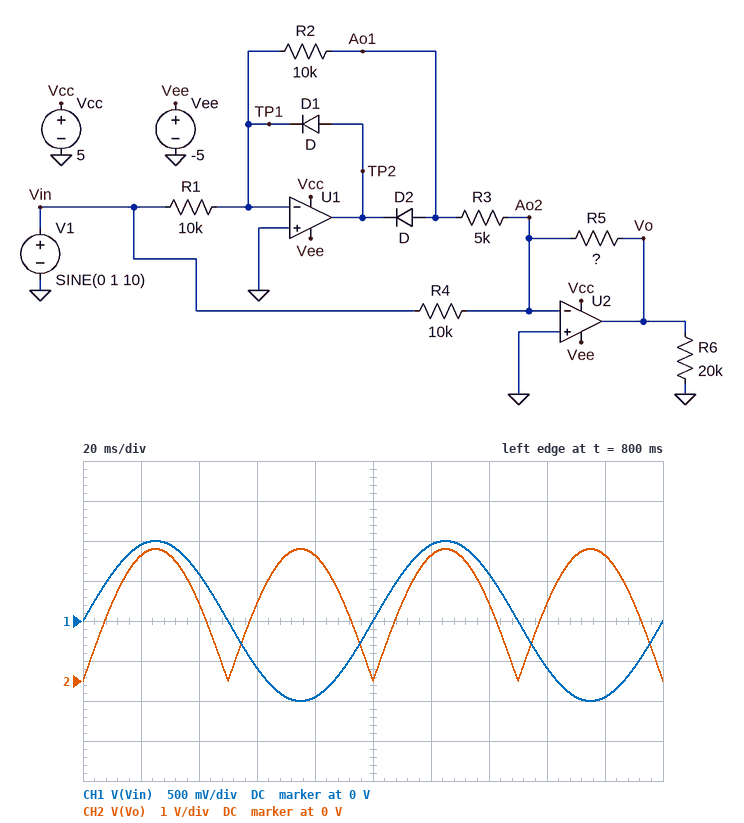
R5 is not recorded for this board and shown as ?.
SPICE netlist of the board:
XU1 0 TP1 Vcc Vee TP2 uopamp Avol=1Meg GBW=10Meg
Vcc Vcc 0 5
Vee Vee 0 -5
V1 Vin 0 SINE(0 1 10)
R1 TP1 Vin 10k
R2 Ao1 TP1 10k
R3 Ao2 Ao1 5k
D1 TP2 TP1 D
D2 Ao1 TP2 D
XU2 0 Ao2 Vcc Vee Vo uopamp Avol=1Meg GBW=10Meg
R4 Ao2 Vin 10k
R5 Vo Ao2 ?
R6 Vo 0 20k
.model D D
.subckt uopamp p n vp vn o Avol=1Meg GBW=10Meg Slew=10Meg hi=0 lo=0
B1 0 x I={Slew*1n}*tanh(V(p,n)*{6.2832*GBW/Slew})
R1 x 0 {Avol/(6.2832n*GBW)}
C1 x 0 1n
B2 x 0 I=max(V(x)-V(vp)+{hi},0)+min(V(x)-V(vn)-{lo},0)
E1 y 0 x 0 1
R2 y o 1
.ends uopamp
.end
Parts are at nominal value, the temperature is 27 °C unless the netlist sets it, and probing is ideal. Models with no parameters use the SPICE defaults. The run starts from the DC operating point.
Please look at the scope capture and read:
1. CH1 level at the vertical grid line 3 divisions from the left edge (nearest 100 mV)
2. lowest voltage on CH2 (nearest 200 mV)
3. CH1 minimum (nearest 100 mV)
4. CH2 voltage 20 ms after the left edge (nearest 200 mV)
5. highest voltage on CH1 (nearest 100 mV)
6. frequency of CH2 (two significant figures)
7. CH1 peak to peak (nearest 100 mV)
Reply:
-600 mV
0 V
-1.0 V
3.2 V
1.0 V
20 Hz
2.0 V
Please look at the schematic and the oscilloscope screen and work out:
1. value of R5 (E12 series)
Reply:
33 kΩ
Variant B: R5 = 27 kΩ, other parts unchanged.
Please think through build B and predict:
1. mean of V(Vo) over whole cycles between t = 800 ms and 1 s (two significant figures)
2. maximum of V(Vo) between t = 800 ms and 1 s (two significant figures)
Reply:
1.7 V
2.7 V
